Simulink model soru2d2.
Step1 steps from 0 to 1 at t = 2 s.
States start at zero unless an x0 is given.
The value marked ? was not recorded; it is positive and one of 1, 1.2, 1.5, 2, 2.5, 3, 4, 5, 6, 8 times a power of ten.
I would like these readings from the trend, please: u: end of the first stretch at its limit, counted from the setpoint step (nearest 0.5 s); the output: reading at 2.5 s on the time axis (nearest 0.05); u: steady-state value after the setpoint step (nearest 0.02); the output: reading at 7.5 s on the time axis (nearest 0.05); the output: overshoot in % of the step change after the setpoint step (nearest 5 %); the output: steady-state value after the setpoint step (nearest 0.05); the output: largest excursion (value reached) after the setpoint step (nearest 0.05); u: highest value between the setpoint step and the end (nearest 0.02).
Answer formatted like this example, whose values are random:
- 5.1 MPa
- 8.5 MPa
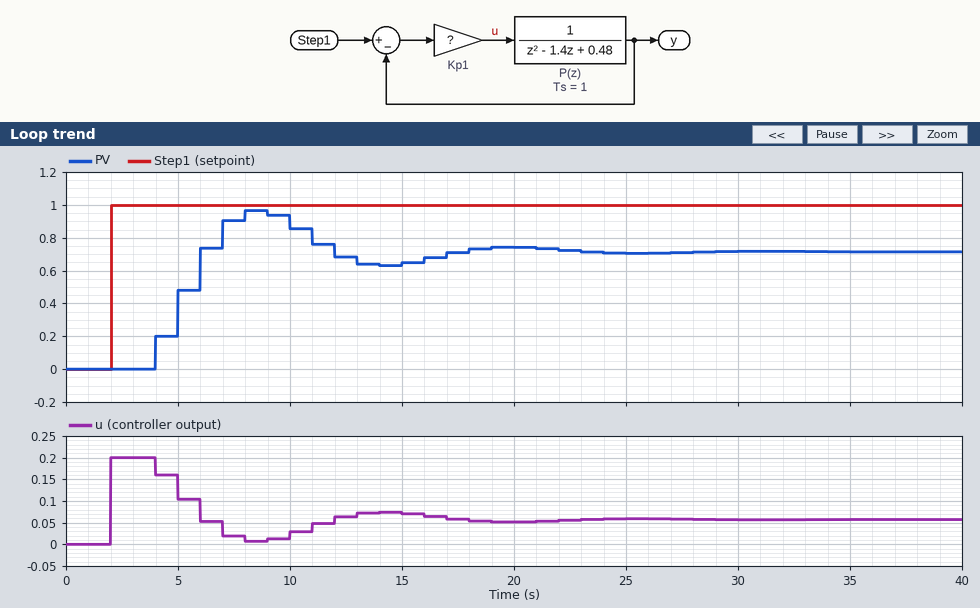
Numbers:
- 2.0 s
- 0.00
- 0.06
- 0.90
- 35 %
- 0.70
- 0.95
- 0.20
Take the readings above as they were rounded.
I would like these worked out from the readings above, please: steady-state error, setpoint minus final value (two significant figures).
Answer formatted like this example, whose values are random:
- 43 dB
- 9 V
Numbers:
- 0.30
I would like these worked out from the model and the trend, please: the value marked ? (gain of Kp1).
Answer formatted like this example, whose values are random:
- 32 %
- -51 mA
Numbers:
- 0.2
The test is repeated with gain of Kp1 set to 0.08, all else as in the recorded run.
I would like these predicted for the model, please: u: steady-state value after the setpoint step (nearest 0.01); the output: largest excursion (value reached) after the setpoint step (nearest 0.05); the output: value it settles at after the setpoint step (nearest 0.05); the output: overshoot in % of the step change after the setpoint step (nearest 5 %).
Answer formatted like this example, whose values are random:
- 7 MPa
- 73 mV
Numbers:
- 0.04
- 0.55
- 0.50
- 10 %
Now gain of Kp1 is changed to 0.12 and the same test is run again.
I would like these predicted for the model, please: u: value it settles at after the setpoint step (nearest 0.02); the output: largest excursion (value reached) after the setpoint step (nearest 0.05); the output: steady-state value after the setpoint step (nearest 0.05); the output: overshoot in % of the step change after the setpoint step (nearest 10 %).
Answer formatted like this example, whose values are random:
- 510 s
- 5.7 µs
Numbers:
- 0.04
- 0.70
- 0.60
- 20 %
